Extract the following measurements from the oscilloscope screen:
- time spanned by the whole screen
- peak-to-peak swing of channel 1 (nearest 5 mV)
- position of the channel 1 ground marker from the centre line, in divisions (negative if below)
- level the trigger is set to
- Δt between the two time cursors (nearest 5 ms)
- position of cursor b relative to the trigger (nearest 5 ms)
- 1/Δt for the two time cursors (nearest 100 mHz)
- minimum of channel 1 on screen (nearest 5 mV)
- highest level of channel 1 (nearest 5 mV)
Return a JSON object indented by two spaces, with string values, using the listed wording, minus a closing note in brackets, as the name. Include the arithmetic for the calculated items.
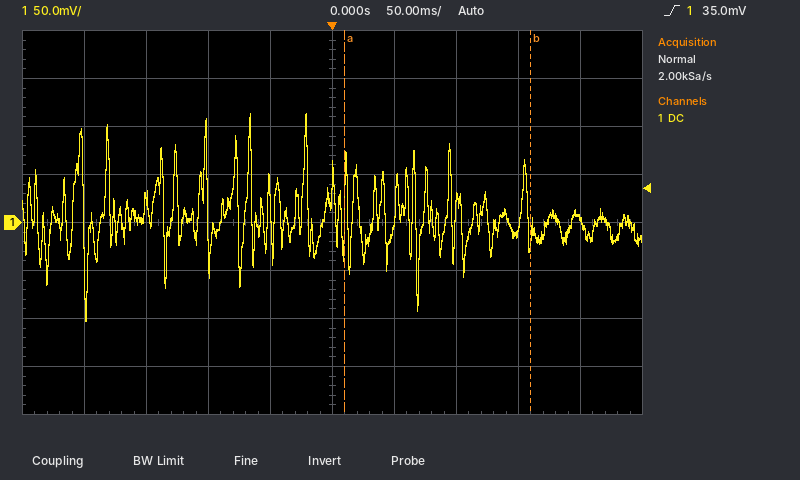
{
  "time spanned by the whole screen": "500 ms",
  "peak-to-peak swing of channel 1": "115 mV − (-100 mV) = 215 mV",
  "position of the channel 1 ground marker from the centre line, in divisions": "0.0 div",
  "level the trigger is set to": "35.0 mV",
  "Δt between the two time cursors": "150 ms",
  "position of cursor b relative to the trigger": "+160 ms",
  "1/Δt for the two time cursors": "1 / 150 ms ≈ 6.7 Hz",
  "minimum of channel 1 on screen": "-100 mV",
  "highest level of channel 1": "115 mV"
}
